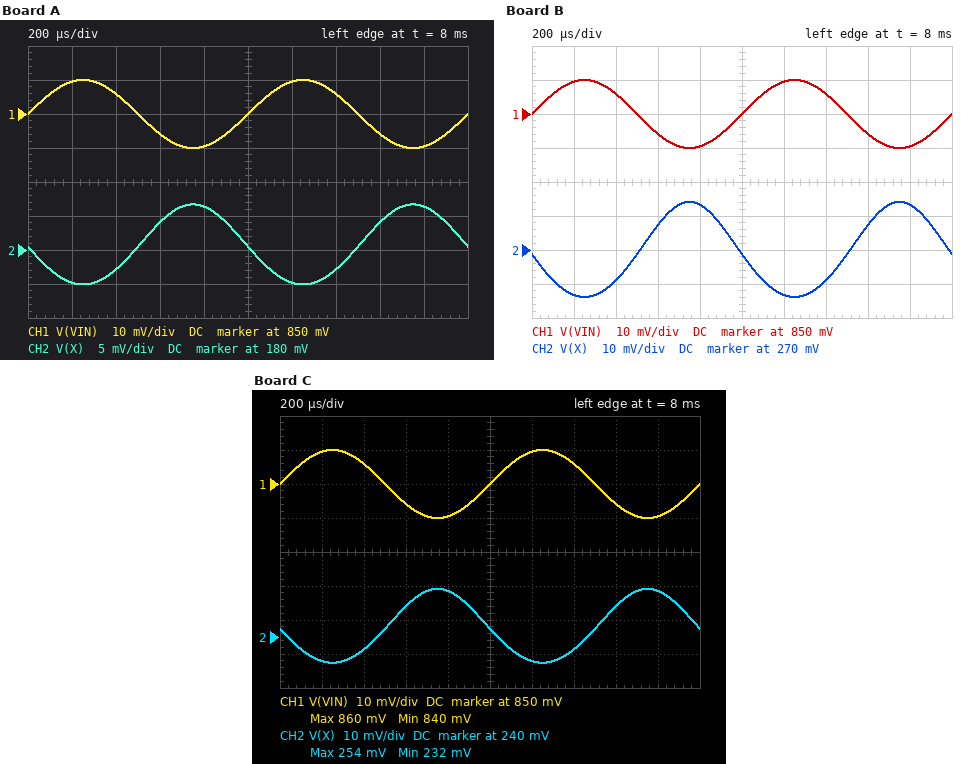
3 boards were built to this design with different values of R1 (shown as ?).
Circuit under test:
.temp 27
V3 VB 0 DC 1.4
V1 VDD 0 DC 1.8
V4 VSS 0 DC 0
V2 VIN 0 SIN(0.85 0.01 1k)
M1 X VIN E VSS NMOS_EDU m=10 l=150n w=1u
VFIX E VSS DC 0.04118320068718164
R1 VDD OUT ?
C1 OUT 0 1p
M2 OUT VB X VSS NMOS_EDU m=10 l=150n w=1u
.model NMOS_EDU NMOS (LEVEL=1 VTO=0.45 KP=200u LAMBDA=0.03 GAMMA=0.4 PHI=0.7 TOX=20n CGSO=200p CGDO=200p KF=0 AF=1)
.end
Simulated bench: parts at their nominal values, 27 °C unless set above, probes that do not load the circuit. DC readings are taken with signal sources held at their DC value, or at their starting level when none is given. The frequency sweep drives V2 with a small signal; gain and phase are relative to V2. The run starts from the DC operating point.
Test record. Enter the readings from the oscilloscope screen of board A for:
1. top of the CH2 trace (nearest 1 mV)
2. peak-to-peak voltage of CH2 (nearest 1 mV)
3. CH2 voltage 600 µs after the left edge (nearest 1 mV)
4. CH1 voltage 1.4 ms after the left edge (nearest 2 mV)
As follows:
187 mV
12 mV
184 mV
856 mV
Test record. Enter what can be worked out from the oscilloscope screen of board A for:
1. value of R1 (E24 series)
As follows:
3 kΩ
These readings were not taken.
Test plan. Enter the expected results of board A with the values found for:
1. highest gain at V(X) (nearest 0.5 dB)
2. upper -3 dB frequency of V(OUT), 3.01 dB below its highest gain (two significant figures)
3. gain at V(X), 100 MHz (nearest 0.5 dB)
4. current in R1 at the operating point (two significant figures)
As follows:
-4.5 dB
370 MHz
-5.0 dB
520 µA
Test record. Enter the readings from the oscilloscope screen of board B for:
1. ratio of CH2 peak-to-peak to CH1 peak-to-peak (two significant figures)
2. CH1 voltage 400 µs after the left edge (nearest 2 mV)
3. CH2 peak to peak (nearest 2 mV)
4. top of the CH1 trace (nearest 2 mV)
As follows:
1.4
856 mV
28 mV
860 mV
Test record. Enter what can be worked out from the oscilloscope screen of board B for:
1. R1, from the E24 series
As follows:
2 kΩ
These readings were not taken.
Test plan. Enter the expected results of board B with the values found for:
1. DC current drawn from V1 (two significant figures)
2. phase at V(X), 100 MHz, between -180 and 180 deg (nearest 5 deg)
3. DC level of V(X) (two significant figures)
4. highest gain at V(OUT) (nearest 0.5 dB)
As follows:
720 µA
165 deg
270 mV
4.0 dB
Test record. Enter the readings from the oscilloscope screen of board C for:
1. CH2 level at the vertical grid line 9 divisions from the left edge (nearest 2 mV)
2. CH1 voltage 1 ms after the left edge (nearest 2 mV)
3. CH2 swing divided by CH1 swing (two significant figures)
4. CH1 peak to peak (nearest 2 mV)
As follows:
254 mV
850 mV
1.1
20 mV
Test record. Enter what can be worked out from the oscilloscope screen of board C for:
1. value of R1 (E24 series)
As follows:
2.2 kΩ
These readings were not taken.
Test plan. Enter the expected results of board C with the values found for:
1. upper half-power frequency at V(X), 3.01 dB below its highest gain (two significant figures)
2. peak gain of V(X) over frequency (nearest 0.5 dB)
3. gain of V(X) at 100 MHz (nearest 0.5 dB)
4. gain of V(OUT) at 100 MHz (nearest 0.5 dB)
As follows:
310 MHz
0.5 dB
0 dB
1.0 dB
